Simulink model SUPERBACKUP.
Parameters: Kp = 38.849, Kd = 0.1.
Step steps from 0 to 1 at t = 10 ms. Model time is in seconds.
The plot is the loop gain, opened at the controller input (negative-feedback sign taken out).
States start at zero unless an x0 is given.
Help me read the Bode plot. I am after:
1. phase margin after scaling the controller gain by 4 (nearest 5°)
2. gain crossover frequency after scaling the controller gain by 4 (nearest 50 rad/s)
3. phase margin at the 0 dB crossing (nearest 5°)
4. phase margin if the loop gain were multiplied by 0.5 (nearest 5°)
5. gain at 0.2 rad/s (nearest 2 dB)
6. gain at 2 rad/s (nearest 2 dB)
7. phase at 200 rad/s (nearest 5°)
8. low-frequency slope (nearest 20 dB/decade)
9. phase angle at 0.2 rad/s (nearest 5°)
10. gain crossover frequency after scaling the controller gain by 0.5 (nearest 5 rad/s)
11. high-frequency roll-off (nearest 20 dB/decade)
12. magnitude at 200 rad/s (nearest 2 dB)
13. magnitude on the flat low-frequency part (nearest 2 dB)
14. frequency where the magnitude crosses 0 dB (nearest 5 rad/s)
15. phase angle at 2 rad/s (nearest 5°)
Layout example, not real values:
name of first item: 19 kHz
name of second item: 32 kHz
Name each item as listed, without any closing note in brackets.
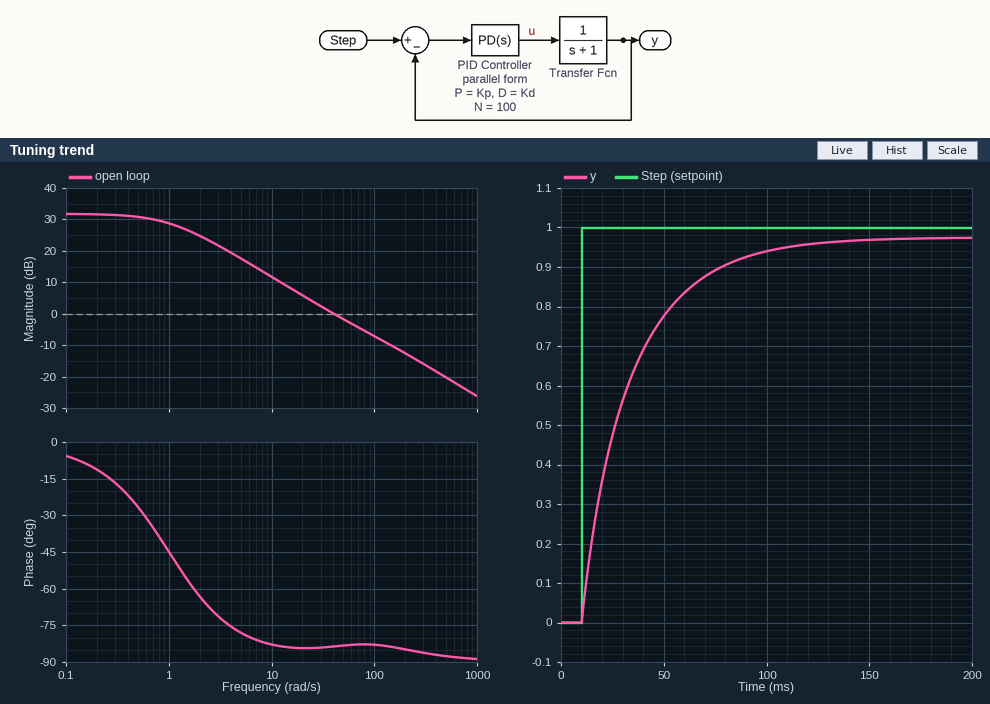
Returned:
phase margin after scaling the controller gain by 4: 95°
gain crossover frequency after scaling the controller gain by 4: 200 rad/s
phase margin at the 0 dB crossing: 95°
phase margin if the loop gain were multiplied by 0.5: 95°
gain at 0.2 rad/s: 32 dB
gain at 2 rad/s: 24 dB
phase at 200 rad/s: -85°
low-frequency slope: 0 dB/decade
phase angle at 0.2 rad/s: -10°
gain crossover frequency after scaling the controller gain by 0.5: 20 rad/s
high-frequency roll-off: -20 dB/decade
magnitude at 200 rad/s: -12 dB
magnitude on the flat low-frequency part: 32 dB
frequency where the magnitude crosses 0 dB: 40 rad/s
phase angle at 2 rad/s: -65°
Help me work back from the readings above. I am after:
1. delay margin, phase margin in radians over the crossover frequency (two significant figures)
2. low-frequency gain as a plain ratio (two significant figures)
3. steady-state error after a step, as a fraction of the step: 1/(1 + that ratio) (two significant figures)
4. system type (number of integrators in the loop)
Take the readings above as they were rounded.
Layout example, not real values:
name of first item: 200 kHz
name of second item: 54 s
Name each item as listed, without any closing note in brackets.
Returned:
delay margin, phase margin in radians over the crossover frequency: 0.041 s
low-frequency gain as a plain ratio: 40
steady-state error after a step, as a fraction of the step: 1/(1 + that ratio): 0.024
system type: 0
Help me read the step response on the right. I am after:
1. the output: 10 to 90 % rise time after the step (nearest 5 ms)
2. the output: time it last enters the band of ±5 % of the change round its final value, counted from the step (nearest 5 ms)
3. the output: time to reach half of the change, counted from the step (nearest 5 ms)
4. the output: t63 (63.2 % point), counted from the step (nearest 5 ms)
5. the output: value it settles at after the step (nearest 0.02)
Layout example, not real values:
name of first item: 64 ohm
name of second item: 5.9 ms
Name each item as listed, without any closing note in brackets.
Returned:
the output: 10 to 90 % rise time after the step: 60 ms
the output: time it last enters the band of ±5 % of the change round its final value, counted from the step: 80 ms
the output: time to reach half of the change, counted from the step: 15 ms
the output: t63 (63.2 % point), counted from the step: 25 ms
the output: value it settles at after the step: 0.98
